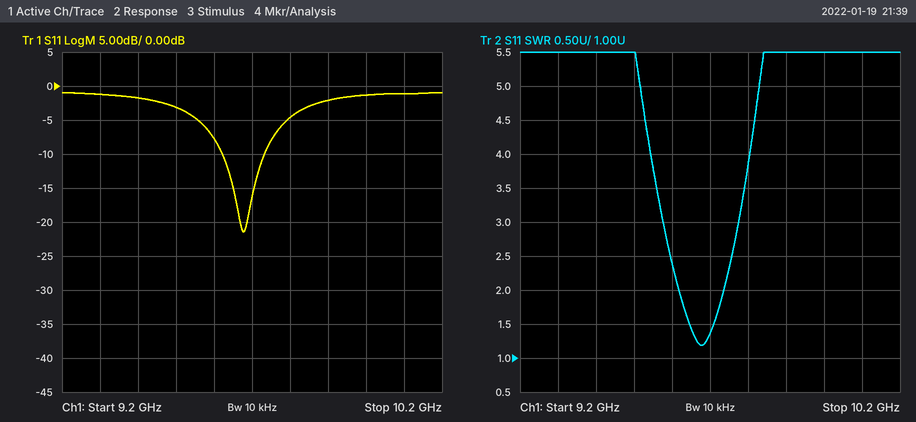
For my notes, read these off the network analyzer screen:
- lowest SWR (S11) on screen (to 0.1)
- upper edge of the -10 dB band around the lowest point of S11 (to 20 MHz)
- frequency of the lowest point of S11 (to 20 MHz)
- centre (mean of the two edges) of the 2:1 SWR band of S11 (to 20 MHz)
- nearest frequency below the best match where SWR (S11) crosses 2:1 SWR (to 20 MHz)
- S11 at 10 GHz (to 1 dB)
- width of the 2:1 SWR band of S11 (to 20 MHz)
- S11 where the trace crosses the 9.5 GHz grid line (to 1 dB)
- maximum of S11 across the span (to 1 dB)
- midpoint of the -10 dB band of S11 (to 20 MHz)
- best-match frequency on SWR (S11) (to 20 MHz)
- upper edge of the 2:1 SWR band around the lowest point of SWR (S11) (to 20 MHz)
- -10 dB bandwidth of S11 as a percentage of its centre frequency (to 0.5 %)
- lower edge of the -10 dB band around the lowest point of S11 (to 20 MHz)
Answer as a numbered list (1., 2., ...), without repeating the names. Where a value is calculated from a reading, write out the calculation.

1. 1.2
2. 9.74 GHz
3. 9.68 GHz
4. 9.68 GHz
5. 9.62 GHz
6. -1 dB
7. 9.74 GHz − 9.62 GHz = 120 MHz
8. -3 dB
9. -1 dB
10. 9.68 GHz
11. 9.68 GHz
12. 9.74 GHz
13. 120 MHz / 9.68 GHz ≈ 1.24 %, so 1.0 % to the nearest 0.5 %
14. 9.62 GHz
